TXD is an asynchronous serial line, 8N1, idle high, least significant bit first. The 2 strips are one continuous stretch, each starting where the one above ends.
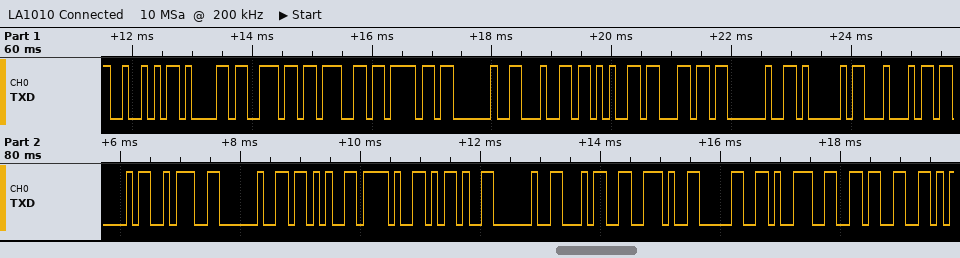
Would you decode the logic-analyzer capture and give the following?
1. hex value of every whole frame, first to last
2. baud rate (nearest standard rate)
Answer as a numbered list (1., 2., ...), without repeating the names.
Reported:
1. 52 61 6E 67 6F 20 64 65 6C 20 41 44 43 3A 20 2B 2F 2D 20 34 2E 30 39 36
2. 9600 baud
